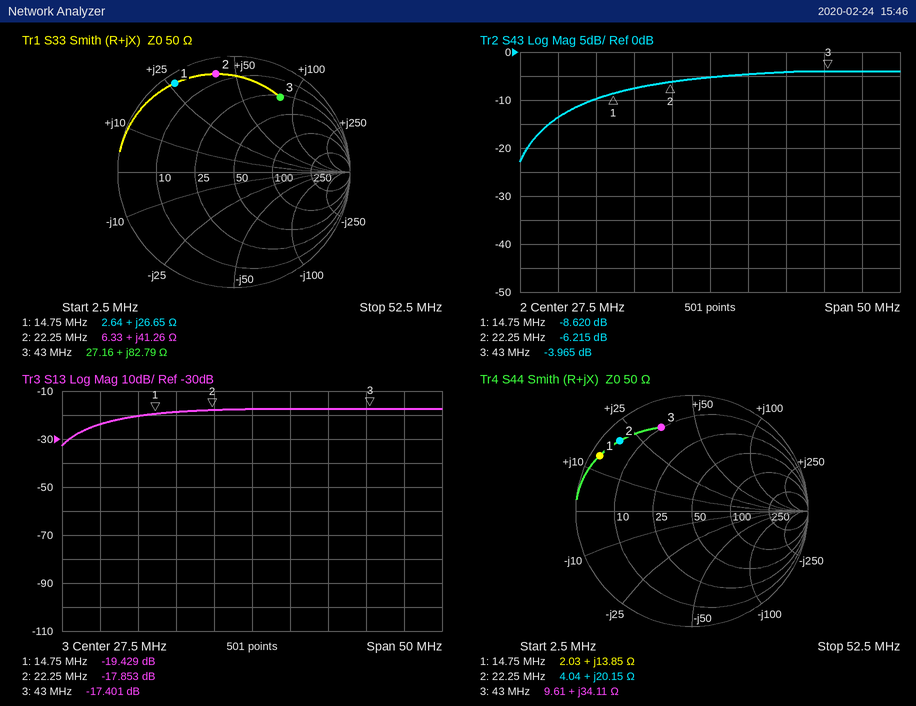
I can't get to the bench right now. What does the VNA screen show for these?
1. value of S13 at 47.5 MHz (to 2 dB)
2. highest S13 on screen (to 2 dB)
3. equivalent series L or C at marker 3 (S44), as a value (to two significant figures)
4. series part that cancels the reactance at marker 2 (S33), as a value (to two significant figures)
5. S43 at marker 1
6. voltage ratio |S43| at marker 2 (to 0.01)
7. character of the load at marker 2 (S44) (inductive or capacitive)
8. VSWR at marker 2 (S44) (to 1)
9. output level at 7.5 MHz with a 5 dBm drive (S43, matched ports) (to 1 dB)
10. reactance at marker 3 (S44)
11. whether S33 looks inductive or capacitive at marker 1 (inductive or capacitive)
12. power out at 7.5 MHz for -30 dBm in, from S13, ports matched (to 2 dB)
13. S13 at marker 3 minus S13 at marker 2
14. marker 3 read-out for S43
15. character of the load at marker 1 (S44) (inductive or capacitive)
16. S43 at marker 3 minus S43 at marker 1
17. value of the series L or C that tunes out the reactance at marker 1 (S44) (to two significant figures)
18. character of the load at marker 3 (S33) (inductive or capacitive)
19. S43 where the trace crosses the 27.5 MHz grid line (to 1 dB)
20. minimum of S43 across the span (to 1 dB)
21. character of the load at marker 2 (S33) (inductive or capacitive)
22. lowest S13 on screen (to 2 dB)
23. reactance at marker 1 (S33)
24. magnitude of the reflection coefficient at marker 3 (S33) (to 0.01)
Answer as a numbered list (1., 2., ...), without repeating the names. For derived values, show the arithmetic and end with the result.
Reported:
1. -18 dB
2. -18 dB
3. L = 34.11 Ω/(2π × 43 MHz) ≈ 126 nH, so 130 nH to two significant figures
4. C = 1/(2π × 22.25 MHz × 41.26 Ω) ≈ 173 pF, so 170 pF to two significant figures
5. -8.620 dB
6. 10^(-6.215/20) ≈ 0.49
7. inductive
8. 14
9. 5 dBm + (-14 dB) = -9 dBm
10. +34.11 Ω
11. inductive
12. -30 dBm + (-24 dB) = -54 dBm
13. -17.401 − (-17.853) = 0.452 dB
14. -3.965 dB
15. inductive
16. -3.965 − (-8.62) = 4.655 dB
17. C = 1/(2π × 14.75 MHz × 13.85 Ω) ≈ 779 pF, so 780 pF to two significant figures
18. inductive
19. -5 dB
20. -23 dB
21. inductive
22. -32 dB
23. +26.65 Ω
24. 0.76
